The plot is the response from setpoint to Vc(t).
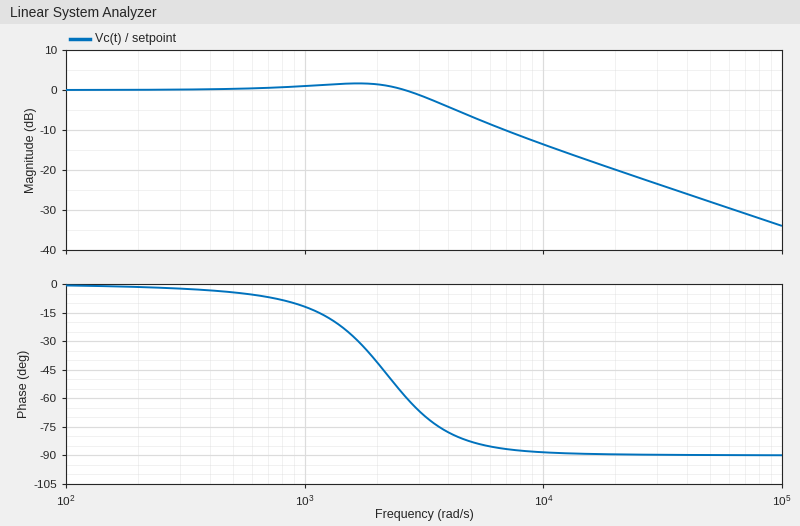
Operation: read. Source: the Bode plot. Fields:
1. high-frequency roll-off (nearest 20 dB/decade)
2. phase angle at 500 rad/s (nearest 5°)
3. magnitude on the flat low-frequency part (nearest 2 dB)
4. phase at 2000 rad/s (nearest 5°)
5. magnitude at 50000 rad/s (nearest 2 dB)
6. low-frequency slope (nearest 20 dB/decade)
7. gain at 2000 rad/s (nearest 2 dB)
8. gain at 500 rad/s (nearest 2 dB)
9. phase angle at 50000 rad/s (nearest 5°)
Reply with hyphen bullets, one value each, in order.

- -20 dB/decade
- -5°
- 0 dB
- -40°
- -28 dB
- 0 dB/decade
- 2 dB
- 0 dB
- -90°
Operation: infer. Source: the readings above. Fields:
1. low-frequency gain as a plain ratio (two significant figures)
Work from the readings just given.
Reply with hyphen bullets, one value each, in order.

- 1.0
